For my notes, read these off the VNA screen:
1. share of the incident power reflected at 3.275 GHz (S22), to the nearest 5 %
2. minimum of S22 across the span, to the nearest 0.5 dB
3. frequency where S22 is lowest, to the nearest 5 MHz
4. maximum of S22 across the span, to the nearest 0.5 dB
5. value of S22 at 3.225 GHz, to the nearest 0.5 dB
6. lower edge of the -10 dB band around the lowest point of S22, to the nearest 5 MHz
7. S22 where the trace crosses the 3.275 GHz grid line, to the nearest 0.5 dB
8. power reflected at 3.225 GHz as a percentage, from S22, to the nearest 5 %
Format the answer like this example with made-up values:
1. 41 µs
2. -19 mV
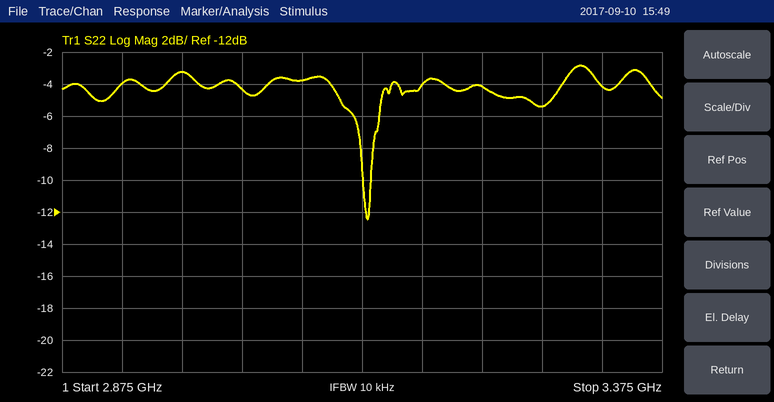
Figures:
1. 30 %
2. -12.5 dB
3. 3.130 GHz
4. -3.0 dB
5. -4.0 dB
6. 3.125 GHz
7. -5.5 dB
8. 40 %
